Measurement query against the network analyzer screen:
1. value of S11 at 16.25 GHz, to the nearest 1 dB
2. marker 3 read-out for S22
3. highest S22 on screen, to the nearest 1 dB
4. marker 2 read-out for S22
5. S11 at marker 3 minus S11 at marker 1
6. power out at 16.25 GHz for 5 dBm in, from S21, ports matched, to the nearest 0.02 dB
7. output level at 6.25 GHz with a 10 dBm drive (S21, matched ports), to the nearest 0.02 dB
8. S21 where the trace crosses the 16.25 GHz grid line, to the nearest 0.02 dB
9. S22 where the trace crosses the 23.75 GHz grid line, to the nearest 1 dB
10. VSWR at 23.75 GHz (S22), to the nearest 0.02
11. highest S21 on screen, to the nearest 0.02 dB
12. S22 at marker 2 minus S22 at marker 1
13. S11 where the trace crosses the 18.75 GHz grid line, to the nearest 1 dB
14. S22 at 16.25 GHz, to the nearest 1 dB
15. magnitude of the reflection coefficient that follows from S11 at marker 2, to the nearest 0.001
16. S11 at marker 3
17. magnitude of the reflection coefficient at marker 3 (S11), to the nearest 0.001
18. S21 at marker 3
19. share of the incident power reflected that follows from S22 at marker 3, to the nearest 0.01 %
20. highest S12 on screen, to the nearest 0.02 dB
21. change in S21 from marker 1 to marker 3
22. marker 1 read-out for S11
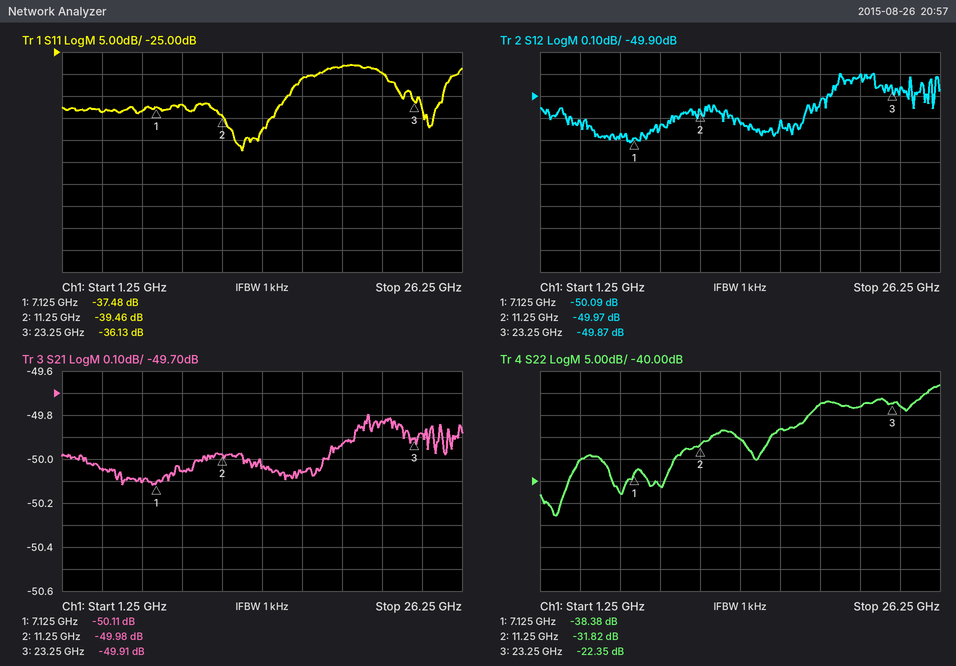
-31 dB
-22.35 dB
-18 dB
-31.82 dB
1.35 dB
-45.06 dBm
-40.10 dBm
-50.06 dB
-23 dB
1.16
-49.80 dB
6.56 dB
-28 dB
-28 dB
0.011
-36.13 dB
0.016
-49.91 dB
0.58 %
-49.80 dB
0.20 dB
-37.48 dB
